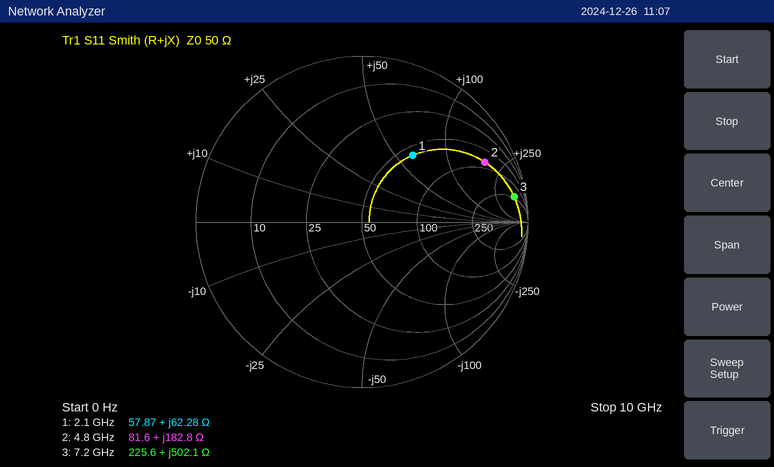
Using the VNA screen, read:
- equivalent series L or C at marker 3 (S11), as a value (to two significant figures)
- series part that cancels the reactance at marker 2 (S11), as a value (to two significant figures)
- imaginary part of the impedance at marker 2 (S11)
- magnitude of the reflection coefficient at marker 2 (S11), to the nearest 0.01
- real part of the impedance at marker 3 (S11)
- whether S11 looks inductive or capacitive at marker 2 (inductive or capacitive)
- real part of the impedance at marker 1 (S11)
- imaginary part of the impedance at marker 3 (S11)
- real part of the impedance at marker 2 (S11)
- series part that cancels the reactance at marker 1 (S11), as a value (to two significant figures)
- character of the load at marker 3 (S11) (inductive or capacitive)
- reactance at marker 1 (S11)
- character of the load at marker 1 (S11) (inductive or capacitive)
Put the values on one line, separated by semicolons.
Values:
11 nH; 180 fF; +182.8 Ω; 0.82; 225.6 Ω; inductive; 57.87 Ω; +502.1 Ω; 81.6 Ω; 1.2 pF; inductive; +62.28 Ω; inductive
